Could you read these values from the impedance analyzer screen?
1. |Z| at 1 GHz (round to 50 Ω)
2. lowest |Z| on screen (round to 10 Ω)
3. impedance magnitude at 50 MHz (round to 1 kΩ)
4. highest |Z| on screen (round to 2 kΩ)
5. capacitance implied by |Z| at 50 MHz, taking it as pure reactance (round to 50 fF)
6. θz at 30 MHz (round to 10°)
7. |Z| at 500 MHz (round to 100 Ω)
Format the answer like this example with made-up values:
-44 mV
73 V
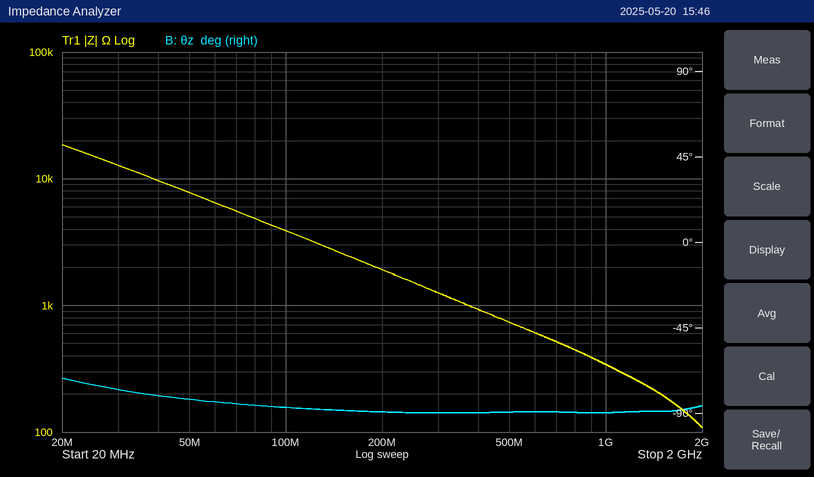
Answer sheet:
350 Ω
110 Ω
8 kΩ
18 kΩ
400 fF
-80°
700 Ω
